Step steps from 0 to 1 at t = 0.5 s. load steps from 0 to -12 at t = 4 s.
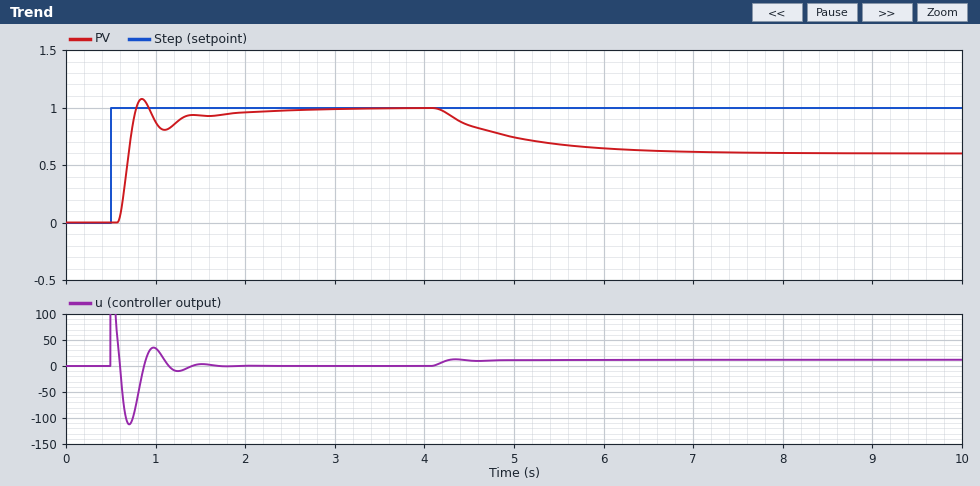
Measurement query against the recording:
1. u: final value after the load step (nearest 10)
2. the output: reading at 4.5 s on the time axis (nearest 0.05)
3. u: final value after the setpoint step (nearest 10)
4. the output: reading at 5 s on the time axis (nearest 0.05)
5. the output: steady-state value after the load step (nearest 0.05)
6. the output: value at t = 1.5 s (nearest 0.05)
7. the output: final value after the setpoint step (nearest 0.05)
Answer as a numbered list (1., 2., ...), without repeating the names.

1. 10
2. 0.85
3. 0
4. 0.75
5. 0.60
6. 0.95
7. 1.00
